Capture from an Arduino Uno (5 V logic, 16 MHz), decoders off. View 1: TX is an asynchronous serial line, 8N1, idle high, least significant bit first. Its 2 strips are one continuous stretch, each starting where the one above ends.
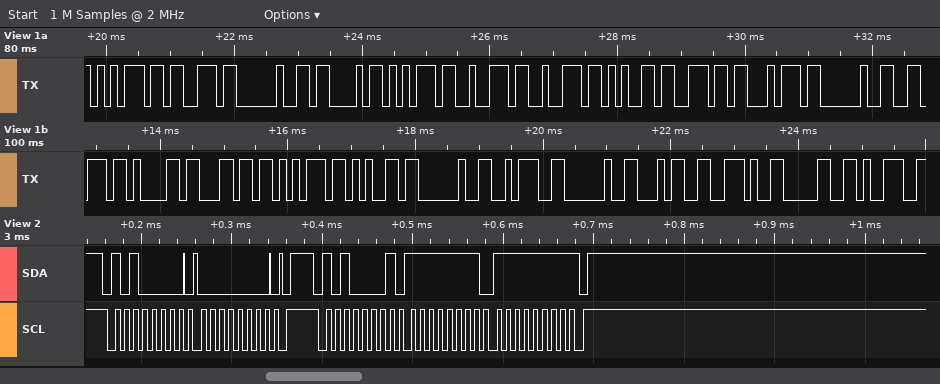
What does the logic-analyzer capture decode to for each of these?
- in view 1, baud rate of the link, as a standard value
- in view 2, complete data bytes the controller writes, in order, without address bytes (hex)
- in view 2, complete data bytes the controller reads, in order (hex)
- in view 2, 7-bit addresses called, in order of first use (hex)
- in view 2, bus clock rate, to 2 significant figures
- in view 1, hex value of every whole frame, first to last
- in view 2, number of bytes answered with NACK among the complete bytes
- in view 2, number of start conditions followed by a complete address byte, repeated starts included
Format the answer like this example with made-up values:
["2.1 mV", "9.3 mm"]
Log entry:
["9600 baud", "00", "FF FF", "0x50", "100 kHz", "0x75 0x73 0x20 0x43 0x75 0x72 0x72 0x65 0x6E 0x74 0x20 0x76 0x61 0x6C 0x75 0x65 0x20 0x3A 0x20 0x34 0x2E 0x30 0x39", "1", "2"]
